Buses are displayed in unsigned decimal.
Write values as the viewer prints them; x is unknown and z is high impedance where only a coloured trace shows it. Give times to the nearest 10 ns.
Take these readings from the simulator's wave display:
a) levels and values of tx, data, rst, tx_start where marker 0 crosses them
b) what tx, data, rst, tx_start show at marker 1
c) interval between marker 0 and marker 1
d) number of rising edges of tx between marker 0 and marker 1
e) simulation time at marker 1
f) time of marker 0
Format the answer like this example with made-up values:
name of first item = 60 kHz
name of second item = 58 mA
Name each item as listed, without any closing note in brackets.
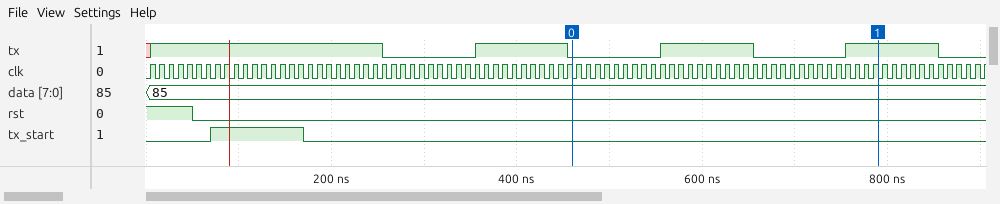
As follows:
levels and values of tx, data, rst, tx_start where marker 0 crosses them = tx=0, data=85, rst=0, tx_start=0
what tx, data, rst, tx_start show at marker 1 = tx=1, data=85, rst=0, tx_start=0
interval between marker 0 and marker 1 = 330 ns
number of rising edges of tx between marker 0 and marker 1 = 2
simulation time at marker 1 = 790 ns
time of marker 0 = 460 ns
